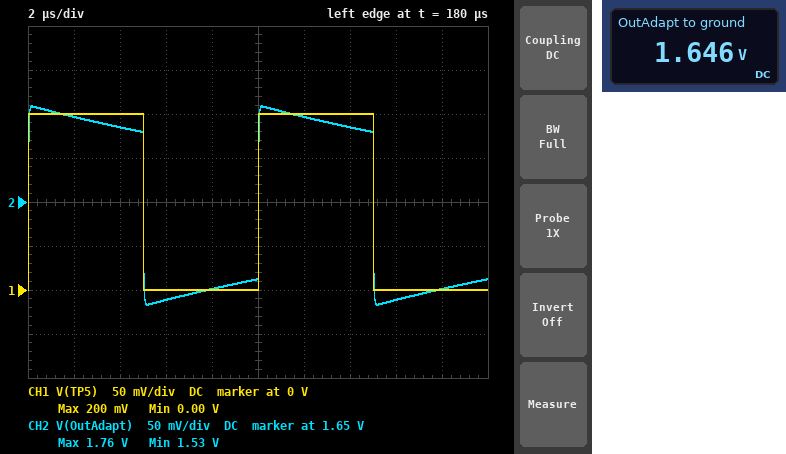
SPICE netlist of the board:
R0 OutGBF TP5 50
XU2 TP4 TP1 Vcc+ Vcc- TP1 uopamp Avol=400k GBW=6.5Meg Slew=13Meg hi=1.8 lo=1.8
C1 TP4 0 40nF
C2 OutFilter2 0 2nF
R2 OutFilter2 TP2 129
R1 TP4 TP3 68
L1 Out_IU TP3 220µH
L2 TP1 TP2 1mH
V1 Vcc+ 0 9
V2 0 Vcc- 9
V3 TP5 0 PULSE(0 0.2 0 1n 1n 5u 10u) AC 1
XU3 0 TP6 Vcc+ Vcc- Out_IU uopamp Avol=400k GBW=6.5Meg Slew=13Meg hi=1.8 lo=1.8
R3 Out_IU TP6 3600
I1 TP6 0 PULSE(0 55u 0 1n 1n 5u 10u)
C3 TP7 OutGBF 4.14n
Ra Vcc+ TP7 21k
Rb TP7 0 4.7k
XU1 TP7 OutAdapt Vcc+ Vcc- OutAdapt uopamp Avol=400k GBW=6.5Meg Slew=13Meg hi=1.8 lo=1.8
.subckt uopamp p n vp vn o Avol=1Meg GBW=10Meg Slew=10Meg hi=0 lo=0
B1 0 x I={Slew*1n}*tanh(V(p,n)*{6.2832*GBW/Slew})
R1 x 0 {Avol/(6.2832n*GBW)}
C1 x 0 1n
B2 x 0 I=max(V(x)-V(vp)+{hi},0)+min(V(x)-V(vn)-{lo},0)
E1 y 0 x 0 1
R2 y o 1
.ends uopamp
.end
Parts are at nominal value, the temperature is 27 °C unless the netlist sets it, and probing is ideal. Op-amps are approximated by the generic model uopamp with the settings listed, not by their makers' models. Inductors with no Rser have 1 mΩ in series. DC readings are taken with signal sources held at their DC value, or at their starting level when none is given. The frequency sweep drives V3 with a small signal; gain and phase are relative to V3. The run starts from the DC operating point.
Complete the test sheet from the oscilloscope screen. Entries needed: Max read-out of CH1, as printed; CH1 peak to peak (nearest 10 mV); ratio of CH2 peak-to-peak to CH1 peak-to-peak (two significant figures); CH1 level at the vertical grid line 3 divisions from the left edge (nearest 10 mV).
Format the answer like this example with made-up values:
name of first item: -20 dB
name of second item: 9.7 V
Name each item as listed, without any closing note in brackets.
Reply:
Max read-out of CH1, as printed: 200 mV
CH1 peak to peak: 200 mV
ratio of CH2 peak-to-peak to CH1 peak-to-peak: 1.1
CH1 level at the vertical grid line 3 divisions from the left edge: 0 V
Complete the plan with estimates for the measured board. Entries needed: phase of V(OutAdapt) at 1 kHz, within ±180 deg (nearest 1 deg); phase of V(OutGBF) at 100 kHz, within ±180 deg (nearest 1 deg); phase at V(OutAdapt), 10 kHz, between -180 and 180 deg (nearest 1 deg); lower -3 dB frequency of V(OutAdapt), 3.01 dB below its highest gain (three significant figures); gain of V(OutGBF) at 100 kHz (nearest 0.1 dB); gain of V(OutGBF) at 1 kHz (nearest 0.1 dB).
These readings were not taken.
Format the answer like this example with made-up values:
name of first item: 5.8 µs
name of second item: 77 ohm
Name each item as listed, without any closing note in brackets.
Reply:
phase of V(OutAdapt) at 1 kHz, within ±180 deg: 84 deg
phase of V(OutGBF) at 100 kHz, within ±180 deg: 0 deg
phase at V(OutAdapt), 10 kHz, between -180 and 180 deg: 45 deg
lower -3 dB frequency of V(OutAdapt), 3.01 dB below its highest gain: 9.85 kHz
gain of V(OutGBF) at 100 kHz: -0.1 dB
gain of V(OutGBF) at 1 kHz: 0 dB
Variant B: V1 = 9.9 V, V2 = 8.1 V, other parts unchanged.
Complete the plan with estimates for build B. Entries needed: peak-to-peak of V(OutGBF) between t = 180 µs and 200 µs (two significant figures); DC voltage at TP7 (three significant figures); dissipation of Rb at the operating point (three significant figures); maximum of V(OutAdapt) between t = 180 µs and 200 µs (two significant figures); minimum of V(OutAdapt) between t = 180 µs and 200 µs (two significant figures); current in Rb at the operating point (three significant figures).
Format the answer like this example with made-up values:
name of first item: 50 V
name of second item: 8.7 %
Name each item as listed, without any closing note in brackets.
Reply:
peak-to-peak of V(OutGBF) between t = 180 µs and 200 µs: 200 mV
DC voltage at TP7: 1.81 V
dissipation of Rb at the operating point: 697 µW
maximum of V(OutAdapt) between t = 180 µs and 200 µs: 1.9 V
minimum of V(OutAdapt) between t = 180 µs and 200 µs: 1.7 V
current in Rb at the operating point: 385 µA
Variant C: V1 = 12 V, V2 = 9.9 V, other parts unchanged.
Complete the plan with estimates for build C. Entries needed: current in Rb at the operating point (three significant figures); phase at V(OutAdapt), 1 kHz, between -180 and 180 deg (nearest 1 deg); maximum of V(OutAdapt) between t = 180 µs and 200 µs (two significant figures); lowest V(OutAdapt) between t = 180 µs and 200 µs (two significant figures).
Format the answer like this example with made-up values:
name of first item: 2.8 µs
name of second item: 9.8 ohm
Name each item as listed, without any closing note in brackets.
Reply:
current in Rb at the operating point: 467 µA
phase at V(OutAdapt), 1 kHz, between -180 and 180 deg: 84 deg
maximum of V(OutAdapt) between t = 180 µs and 200 µs: 2.3 V
lowest V(OutAdapt) between t = 180 µs and 200 µs: 2.1 V
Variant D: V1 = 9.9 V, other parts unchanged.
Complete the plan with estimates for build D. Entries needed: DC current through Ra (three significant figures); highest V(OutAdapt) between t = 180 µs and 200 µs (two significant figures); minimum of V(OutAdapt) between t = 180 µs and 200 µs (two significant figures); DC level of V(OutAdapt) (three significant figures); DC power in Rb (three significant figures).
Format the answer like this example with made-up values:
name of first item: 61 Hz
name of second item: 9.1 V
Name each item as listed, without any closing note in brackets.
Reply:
DC current through Ra: 385 µA
highest V(OutAdapt) between t = 180 µs and 200 µs: 1.9 V
minimum of V(OutAdapt) between t = 180 µs and 200 µs: 1.7 V
DC level of V(OutAdapt): 1.81 V
DC power in Rb: 697 µW
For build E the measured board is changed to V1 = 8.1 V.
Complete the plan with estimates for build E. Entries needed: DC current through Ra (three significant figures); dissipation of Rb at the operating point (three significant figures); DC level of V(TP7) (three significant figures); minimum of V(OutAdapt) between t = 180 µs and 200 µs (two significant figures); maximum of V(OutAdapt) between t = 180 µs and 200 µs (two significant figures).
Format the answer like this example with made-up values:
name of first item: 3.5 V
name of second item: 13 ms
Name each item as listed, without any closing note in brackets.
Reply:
DC current through Ra: 315 µA
dissipation of Rb at the operating point: 467 µW
DC level of V(TP7): 1.48 V
minimum of V(OutAdapt) between t = 180 µs and 200 µs: 1.4 V
maximum of V(OutAdapt) between t = 180 µs and 200 µs: 1.6 V
